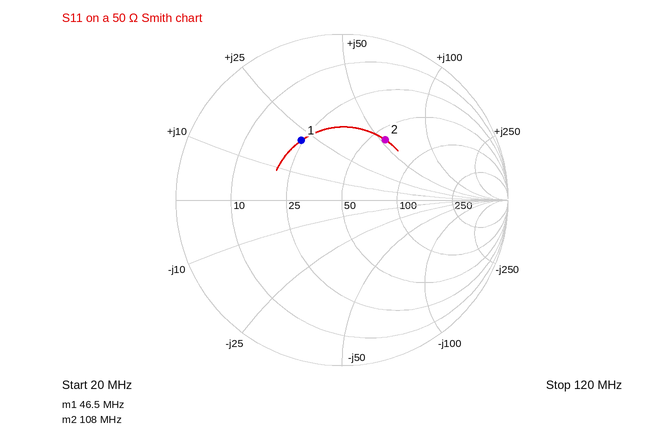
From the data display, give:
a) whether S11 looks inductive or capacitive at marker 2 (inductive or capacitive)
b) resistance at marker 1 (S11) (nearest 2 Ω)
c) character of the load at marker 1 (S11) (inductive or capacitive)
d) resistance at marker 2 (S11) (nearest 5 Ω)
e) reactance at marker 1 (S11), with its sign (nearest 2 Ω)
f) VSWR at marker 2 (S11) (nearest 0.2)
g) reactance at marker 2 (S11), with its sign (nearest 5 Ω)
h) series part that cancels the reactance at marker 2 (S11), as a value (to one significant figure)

inductive
24 Ω
inductive
60 Ω
+22 Ω
2.6
+55 Ω
30 pF
